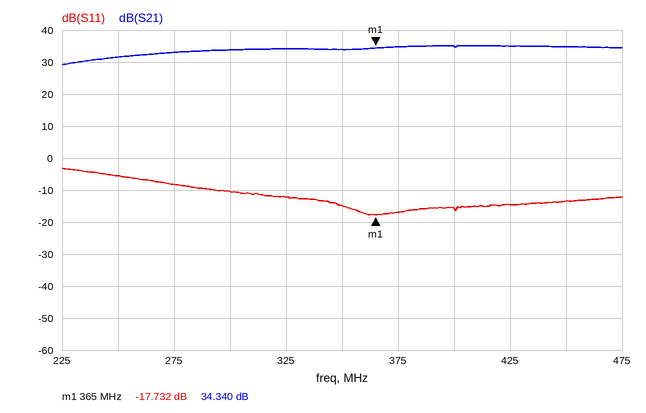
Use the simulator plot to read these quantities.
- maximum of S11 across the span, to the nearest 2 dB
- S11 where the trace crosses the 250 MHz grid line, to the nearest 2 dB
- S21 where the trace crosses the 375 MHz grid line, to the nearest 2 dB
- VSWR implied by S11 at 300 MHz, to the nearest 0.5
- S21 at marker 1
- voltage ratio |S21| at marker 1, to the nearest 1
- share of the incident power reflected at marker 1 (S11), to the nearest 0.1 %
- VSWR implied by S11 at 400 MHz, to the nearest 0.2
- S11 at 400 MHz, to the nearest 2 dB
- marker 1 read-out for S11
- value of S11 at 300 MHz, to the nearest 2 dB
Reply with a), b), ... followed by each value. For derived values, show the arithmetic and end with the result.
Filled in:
a) -4 dB
b) -6 dB
c) 34 dB
d) |Γ| = 10^(-10/20) = 0.3162; VSWR = (1 + 0.3162)/(1 − 0.3162) ≈ 1.92, so 2.0 to the nearest 0.5
e) 34.340 dB
f) 10^(34.34/20) ≈ 52
g) 10^(-17.732/10) ≈ 1.7 %
h) |Γ| = 10^(-16/20) = 0.1585; VSWR = (1 + 0.1585)/(1 − 0.1585) ≈ 1.4
i) -16 dB
j) -17.732 dB
k) -10 dB
